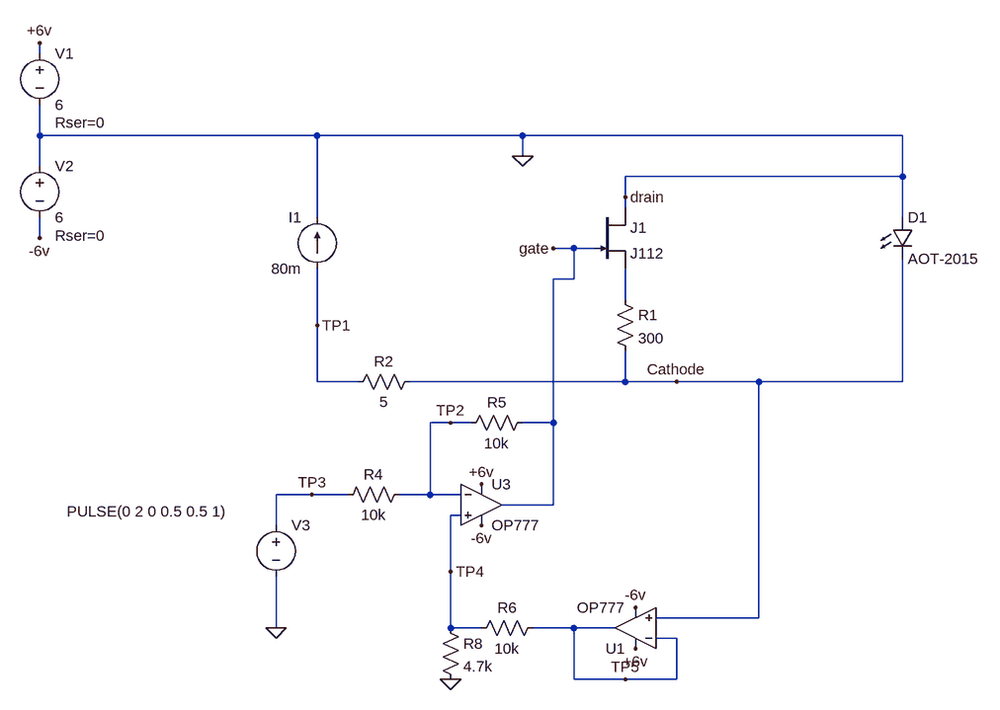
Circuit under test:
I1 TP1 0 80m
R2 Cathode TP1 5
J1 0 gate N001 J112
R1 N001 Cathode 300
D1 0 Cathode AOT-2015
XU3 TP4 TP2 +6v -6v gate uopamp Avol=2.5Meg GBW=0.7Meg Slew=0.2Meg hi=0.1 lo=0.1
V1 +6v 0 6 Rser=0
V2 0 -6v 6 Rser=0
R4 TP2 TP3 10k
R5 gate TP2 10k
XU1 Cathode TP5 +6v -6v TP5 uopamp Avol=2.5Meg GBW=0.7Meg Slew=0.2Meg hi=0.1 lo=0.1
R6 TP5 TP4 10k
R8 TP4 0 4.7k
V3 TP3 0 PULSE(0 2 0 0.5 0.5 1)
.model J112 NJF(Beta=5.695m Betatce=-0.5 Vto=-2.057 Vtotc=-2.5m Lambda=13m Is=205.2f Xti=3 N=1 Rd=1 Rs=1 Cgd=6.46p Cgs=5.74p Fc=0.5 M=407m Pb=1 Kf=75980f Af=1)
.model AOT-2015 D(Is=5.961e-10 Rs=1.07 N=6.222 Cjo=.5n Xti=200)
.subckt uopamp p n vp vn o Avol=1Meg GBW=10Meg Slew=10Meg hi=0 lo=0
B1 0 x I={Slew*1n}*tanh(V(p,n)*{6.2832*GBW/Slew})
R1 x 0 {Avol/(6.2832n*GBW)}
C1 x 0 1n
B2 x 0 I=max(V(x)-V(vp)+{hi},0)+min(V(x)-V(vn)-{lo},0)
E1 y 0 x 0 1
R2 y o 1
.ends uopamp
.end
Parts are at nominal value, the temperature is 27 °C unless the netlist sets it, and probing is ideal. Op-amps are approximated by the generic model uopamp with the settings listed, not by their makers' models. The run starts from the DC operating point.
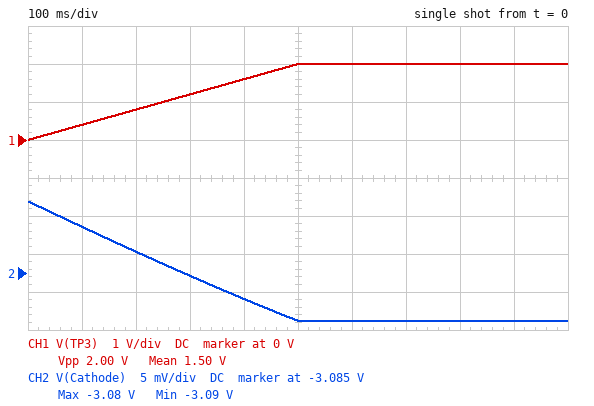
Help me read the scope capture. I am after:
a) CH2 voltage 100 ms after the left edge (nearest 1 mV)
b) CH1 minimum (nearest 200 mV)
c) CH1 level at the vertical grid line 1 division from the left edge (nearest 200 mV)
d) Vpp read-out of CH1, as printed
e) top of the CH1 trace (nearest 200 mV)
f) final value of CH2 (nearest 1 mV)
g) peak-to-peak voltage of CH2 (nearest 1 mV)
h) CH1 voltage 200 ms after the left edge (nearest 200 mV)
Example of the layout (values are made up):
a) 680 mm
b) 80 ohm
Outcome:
a) -3.079 V
b) 0 V
c) 400 mV
d) 2.00 V
e) 2.0 V
f) -3.091 V
g) 16 mV
h) 800 mV
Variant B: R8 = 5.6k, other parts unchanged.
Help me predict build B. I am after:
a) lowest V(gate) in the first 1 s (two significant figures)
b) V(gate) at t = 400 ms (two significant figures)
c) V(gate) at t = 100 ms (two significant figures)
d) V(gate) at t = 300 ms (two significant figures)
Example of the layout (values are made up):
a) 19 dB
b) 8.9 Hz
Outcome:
a) -4.2 V
b) -3.8 V
c) -2.6 V
d) -3.4 V
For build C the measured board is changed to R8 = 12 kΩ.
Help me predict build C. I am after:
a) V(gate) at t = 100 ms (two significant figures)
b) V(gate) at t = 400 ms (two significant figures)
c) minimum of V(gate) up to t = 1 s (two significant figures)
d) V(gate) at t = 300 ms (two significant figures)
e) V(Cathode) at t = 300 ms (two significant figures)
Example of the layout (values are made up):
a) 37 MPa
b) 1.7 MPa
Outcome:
a) -3.8 V
b) -5.0 V
c) -5.4 V
d) -4.6 V
e) -3.1 V
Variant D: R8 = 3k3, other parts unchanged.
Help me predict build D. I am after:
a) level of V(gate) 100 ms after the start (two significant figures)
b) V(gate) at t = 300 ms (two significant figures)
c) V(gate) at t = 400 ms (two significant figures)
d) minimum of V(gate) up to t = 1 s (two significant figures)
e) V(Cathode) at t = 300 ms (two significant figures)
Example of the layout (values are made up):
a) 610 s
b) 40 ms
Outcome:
a) -1.9 V
b) -2.7 V
c) -3.1 V
d) -3.5 V
e) -3.1 V
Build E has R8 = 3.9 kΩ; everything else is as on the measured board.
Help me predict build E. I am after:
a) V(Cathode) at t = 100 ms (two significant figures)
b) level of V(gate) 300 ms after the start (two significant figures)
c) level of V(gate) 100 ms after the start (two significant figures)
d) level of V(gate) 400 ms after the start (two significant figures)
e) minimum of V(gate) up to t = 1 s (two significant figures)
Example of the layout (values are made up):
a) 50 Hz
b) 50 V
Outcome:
a) -3.1 V
b) -2.9 V
c) -2.1 V
d) -3.3 V
e) -3.7 V
